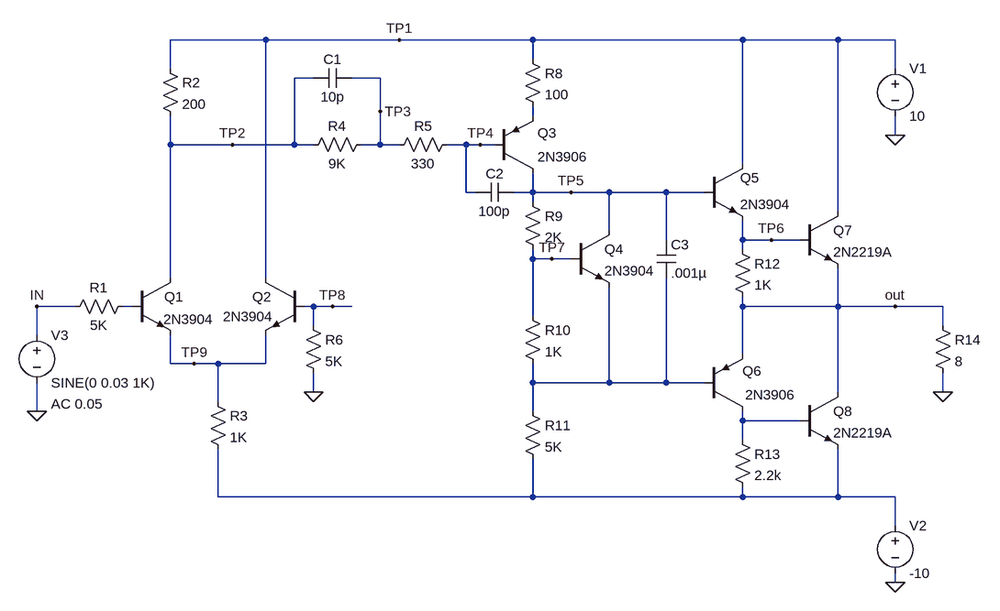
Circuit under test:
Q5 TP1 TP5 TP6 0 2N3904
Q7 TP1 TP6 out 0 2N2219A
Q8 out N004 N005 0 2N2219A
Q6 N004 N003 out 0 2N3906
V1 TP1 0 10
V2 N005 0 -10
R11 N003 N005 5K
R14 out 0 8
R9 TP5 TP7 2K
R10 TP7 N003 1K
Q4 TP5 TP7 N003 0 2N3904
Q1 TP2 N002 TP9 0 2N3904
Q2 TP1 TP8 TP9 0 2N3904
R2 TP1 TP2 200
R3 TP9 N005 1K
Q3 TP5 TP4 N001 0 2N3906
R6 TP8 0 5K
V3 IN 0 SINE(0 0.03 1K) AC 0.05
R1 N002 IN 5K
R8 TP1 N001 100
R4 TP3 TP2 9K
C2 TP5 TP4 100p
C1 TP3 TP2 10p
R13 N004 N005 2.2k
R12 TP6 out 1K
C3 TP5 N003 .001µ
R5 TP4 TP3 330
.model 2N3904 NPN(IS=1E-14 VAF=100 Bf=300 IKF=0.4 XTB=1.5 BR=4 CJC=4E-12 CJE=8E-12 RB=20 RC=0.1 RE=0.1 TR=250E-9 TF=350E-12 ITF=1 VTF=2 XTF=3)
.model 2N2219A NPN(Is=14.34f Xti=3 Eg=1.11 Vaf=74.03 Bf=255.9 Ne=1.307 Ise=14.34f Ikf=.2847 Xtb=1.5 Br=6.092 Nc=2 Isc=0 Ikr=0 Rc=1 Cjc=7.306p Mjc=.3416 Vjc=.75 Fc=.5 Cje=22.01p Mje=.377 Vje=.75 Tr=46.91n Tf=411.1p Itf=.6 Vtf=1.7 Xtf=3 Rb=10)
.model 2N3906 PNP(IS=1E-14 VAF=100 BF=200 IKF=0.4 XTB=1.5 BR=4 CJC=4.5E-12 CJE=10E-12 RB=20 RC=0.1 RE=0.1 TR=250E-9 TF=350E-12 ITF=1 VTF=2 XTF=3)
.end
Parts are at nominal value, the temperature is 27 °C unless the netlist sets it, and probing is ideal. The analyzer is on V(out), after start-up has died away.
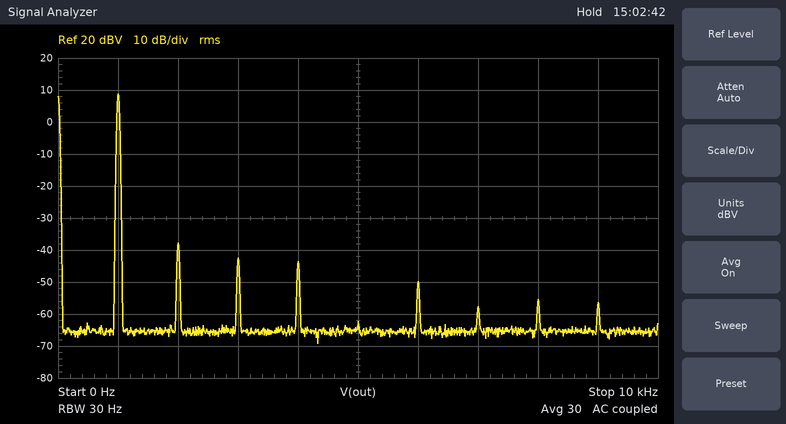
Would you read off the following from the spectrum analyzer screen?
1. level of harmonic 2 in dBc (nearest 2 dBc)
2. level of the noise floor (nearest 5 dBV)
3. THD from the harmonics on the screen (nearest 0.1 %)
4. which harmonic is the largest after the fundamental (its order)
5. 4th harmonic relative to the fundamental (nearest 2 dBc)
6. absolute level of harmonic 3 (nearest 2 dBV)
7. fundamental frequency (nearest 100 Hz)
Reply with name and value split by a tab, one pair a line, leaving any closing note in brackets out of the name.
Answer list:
level of harmonic 2 in dBc	-46 dBc
level of the noise floor	-65 dBV
THD from the harmonics on the screen	0.6 %
which harmonic is the largest after the fundamental	2
4th harmonic relative to the fundamental	-52 dBc
absolute level of harmonic 3	-42 dBV
fundamental frequency	1.0 kHz
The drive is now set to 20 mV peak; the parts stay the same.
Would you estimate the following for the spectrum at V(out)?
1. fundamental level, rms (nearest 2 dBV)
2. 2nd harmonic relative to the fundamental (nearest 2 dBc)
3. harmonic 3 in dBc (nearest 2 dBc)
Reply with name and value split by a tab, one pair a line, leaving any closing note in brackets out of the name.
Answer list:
fundamental level, rms	6 dBV
2nd harmonic relative to the fundamental	-54 dBc
harmonic 3 in dBc	-58 dBc
